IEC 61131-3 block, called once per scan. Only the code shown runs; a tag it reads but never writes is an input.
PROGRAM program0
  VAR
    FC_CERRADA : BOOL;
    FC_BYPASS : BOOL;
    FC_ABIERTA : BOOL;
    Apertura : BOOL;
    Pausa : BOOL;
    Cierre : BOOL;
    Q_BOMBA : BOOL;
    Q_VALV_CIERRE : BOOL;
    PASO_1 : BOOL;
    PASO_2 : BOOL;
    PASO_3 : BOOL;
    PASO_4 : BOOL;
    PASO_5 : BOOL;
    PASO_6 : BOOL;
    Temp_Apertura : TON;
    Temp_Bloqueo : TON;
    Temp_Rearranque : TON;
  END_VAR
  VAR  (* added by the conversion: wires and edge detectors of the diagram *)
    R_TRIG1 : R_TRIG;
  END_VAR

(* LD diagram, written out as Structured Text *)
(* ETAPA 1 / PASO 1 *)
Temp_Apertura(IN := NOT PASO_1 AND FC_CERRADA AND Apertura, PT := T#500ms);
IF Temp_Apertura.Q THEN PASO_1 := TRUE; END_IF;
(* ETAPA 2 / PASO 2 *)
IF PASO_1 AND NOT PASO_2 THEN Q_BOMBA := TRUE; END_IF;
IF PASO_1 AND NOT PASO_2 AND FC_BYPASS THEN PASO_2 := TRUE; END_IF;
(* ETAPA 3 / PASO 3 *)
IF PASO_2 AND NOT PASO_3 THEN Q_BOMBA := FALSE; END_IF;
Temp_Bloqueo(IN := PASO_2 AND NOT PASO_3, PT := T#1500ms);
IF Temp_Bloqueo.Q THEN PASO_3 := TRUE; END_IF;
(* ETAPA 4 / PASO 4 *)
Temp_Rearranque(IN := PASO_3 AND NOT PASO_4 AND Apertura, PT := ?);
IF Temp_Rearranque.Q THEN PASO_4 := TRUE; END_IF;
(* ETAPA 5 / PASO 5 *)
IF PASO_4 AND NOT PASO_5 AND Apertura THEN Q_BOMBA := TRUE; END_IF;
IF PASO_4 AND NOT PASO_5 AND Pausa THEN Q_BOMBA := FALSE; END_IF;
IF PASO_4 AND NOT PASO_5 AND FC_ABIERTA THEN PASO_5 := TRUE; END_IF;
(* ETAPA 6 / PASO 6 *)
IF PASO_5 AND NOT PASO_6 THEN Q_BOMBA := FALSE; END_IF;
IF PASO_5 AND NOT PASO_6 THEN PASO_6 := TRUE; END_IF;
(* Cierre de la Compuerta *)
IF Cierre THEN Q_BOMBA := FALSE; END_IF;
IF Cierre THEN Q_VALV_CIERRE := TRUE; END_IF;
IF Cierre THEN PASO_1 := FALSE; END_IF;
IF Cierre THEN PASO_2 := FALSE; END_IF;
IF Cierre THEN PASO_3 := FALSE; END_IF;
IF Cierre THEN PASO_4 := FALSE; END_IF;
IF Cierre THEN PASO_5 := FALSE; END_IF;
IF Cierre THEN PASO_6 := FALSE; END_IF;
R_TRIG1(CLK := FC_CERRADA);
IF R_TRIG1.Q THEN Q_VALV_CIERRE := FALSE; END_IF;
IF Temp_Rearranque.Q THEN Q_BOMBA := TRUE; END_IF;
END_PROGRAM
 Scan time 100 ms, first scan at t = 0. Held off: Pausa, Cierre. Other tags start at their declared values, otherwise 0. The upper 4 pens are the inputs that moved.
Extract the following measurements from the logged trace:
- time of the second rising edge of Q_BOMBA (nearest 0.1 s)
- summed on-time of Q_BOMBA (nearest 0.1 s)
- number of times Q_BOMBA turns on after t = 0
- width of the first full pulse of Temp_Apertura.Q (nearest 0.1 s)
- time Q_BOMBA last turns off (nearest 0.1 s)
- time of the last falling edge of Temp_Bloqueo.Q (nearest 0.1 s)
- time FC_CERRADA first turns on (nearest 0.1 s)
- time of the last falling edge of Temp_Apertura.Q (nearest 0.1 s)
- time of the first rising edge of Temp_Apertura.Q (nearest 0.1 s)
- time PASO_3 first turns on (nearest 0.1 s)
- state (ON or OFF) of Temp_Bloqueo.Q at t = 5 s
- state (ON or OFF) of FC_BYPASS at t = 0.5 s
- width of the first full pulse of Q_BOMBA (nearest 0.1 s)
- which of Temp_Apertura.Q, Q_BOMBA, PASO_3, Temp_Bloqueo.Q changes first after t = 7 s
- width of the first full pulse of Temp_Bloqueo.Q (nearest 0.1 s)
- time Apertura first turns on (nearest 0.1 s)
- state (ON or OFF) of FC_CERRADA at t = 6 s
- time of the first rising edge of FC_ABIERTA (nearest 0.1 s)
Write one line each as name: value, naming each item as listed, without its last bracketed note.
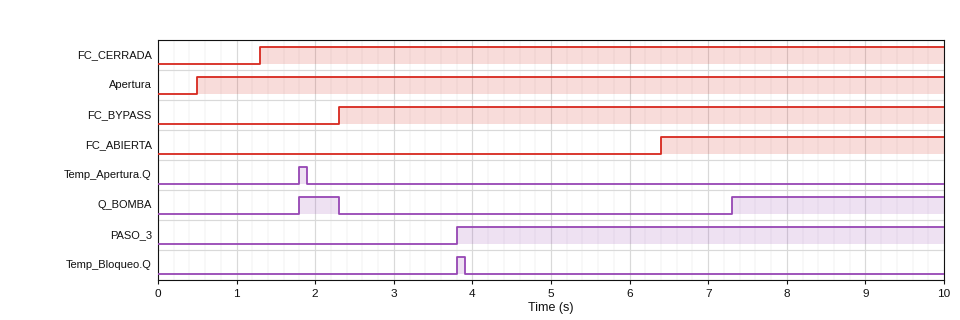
time of the second rising edge of Q_BOMBA: 7.3 s
summed on-time of Q_BOMBA: 3.2 s
number of times Q_BOMBA turns on after t = 0: 2
width of the first full pulse of Temp_Apertura.Q: 0.1 s
time Q_BOMBA last turns off: 2.3 s
time of the last falling edge of Temp_Bloqueo.Q: 3.9 s
time FC_CERRADA first turns on: 1.3 s
time of the last falling edge of Temp_Apertura.Q: 1.9 s
time of the first rising edge of Temp_Apertura.Q: 1.8 s
time PASO_3 first turns on: 3.8 s
state (ON or OFF) of Temp_Bloqueo.Q at t = 5 s: OFF
state (ON or OFF) of FC_BYPASS at t = 0.5 s: OFF
width of the first full pulse of Q_BOMBA: 0.5 s
which of Temp_Apertura.Q, Q_BOMBA, PASO_3, Temp_Bloqueo.Q changes first after t = 7 s: Q_BOMBA
width of the first full pulse of Temp_Bloqueo.Q: 0.1 s
time Apertura first turns on: 0.5 s
state (ON or OFF) of FC_CERRADA at t = 6 s: ON
time of the first rising edge of FC_ABIERTA: 6.4 s
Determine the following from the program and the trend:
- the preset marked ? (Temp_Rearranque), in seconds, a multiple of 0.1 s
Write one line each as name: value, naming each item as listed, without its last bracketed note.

the preset marked ? (Temp_Rearranque), in seconds, a multiple of 0.1 s: 3.5 s
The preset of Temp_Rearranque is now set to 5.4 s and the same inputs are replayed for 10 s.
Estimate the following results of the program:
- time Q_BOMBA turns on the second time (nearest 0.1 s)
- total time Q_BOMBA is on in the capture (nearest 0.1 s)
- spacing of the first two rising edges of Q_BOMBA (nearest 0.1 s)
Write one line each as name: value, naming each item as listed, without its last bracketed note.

time Q_BOMBA turns on the second time: 9.2 s
total time Q_BOMBA is on in the capture: 1.3 s
spacing of the first two rising edges of Q_BOMBA: 7.4 s
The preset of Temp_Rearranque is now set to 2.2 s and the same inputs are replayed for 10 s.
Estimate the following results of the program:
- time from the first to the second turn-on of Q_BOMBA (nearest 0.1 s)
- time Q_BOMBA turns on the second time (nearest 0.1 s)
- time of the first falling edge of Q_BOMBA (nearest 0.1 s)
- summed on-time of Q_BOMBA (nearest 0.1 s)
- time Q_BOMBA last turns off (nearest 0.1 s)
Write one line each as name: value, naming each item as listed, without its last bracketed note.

time from the first to the second turn-on of Q_BOMBA: 4.2 s
time Q_BOMBA turns on the second time: 6.0 s
time of the first falling edge of Q_BOMBA: 2.3 s
summed on-time of Q_BOMBA: 0.9 s
time Q_BOMBA last turns off: 6.4 s
